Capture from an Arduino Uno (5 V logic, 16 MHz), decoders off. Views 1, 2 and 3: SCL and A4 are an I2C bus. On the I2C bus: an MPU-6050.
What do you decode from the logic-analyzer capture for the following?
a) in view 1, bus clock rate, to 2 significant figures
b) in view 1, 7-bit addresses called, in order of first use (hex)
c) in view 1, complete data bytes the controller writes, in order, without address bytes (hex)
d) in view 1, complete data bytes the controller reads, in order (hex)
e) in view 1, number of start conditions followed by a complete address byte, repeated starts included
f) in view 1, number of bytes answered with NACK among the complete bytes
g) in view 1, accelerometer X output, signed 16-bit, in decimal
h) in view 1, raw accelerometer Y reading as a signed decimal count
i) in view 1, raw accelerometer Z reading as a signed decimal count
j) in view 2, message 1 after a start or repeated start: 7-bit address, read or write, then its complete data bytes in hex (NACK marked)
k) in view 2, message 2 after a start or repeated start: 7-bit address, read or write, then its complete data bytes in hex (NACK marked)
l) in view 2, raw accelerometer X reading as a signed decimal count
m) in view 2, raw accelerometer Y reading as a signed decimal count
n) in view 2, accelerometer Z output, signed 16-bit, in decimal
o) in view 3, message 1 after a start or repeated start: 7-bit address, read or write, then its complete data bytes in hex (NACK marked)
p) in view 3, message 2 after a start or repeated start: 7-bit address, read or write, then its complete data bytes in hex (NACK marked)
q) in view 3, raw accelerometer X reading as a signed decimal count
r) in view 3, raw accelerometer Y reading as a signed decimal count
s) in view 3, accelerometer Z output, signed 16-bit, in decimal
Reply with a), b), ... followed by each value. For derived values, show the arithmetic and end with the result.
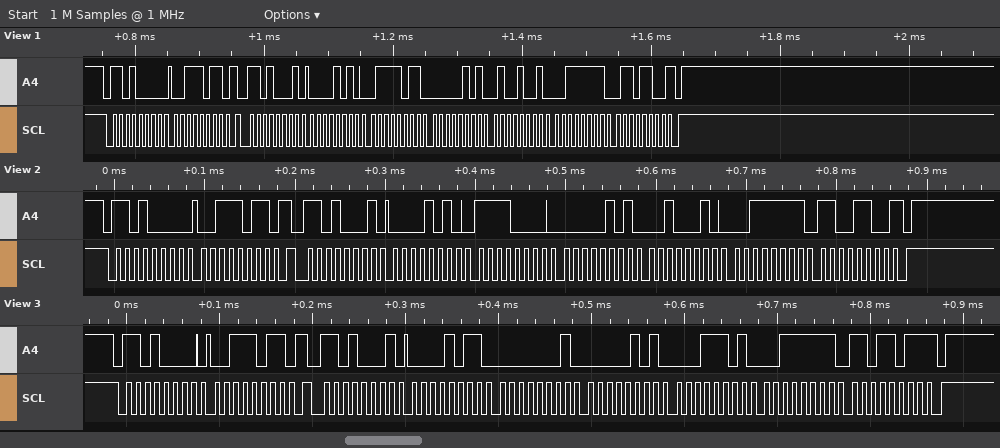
a) 100 kHz
b) 0x68
c) 3B
d) 0A 7B 05 49 3F 6C
e) 2
f) 1
g) 0x0A7B = 2683
h) 0x0549 = 1353
i) 0x3F6C = 16236
j) 0x68 write: 3B
k) 0x68 read: 0A F0 05 22 3F CC NACK
l) 0x0AF0 = 2800
m) 0x0522 = 1314
n) 0x3FCC = 16332
o) 0x68 write: 3B
p) 0x68 read: 0B 01 05 1D 3F DB NACK
q) 0x0B01 = 2817
r) 0x051D = 1309
s) 0x3FDB = 16347
